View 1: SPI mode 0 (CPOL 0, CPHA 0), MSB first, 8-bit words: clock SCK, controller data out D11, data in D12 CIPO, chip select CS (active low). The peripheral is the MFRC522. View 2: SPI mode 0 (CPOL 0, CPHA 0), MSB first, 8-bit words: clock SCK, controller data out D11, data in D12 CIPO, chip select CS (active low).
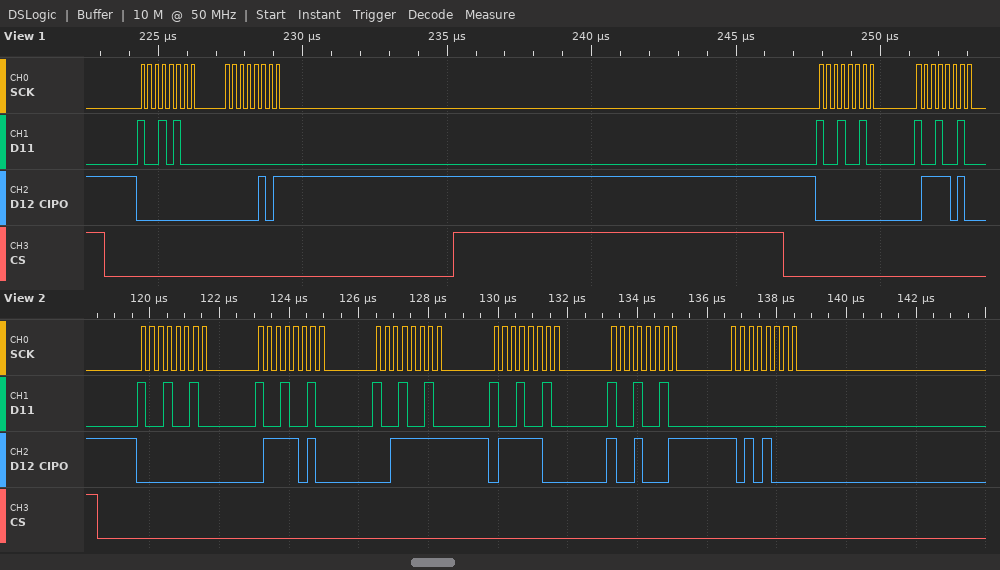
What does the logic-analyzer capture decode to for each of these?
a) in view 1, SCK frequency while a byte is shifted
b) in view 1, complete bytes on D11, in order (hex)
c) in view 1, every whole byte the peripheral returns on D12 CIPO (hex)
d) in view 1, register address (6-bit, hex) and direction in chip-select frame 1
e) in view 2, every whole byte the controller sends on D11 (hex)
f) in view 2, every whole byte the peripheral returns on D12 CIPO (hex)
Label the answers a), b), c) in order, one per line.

a) 4 MHz
b) 0x94 0x00 0x92 0x92
c) 0x00 0x05 0x00 0x7A
d) 0x0A read
e) 92 92 92 92 92 00
f) 00 7A 3F 7C 91 A8
